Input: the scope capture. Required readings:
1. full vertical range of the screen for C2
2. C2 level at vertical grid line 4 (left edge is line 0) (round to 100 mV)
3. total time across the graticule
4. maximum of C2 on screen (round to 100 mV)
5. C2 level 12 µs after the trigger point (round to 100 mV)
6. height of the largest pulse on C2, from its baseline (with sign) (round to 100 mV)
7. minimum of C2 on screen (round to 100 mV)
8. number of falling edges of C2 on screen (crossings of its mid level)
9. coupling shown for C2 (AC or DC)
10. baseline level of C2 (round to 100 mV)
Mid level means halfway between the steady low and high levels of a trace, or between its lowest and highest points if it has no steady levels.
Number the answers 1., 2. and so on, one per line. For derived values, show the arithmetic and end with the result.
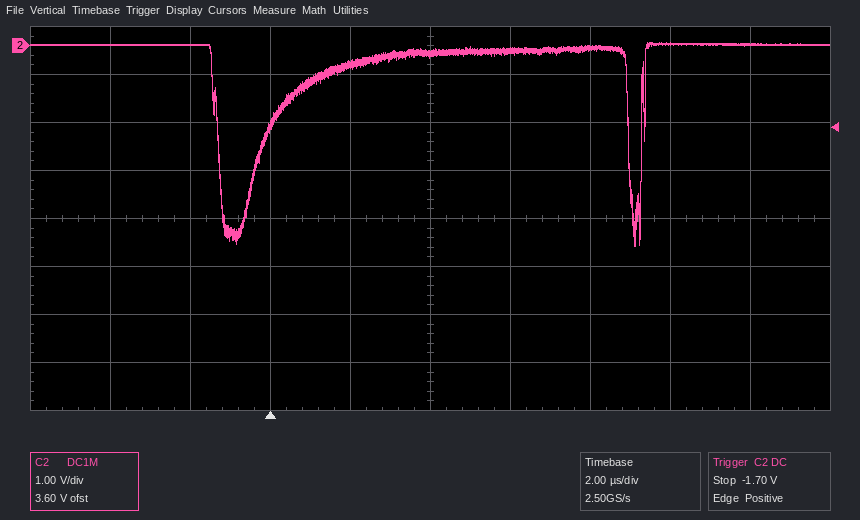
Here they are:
1. 8 V
2. -400 mV
3. 20 µs
4. 100 mV
5. 0.0 V
6. -4.2 V − (0.0 V) = -4.2 V
7. -4.2 V
8. 2
9. DC
10. 0.0 V
